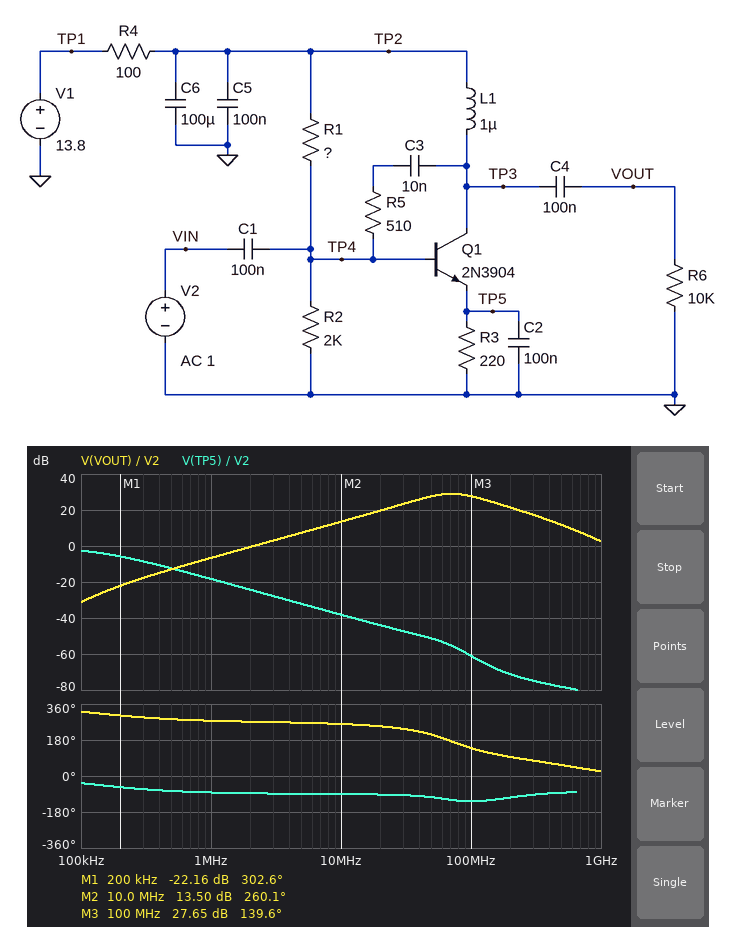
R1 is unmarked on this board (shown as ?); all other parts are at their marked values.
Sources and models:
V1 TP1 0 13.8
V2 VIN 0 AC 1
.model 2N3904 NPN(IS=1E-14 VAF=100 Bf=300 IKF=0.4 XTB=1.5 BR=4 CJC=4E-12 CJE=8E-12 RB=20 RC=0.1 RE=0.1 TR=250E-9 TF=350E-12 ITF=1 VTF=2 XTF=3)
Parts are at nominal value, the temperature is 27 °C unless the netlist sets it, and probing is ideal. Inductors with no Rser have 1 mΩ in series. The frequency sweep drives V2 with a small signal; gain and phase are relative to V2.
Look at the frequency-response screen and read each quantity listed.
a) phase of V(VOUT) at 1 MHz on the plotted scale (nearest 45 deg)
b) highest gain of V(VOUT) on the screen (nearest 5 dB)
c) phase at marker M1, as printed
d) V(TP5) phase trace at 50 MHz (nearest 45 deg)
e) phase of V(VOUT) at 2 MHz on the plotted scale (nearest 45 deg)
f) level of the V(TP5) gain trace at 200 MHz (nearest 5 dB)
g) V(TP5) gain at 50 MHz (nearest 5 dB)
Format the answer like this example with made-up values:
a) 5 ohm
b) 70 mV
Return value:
a) 270 deg
b) 30 dB
c) 302.6 deg
d) -90 deg
e) 270 deg
f) -70 dB
g) -50 dB
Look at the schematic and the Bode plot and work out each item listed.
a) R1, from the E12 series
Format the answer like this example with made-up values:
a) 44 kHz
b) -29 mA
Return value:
a) 22 kΩ
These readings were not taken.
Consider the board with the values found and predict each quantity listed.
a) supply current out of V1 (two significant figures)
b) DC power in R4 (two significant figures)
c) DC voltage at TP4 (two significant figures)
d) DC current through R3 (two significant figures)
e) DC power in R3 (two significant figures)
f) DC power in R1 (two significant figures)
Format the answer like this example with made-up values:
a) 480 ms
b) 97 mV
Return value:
a) 2.6 mA
b) 670 µW
c) 1.1 V
d) 2.0 mA
e) 910 µW
f) 7.0 mW
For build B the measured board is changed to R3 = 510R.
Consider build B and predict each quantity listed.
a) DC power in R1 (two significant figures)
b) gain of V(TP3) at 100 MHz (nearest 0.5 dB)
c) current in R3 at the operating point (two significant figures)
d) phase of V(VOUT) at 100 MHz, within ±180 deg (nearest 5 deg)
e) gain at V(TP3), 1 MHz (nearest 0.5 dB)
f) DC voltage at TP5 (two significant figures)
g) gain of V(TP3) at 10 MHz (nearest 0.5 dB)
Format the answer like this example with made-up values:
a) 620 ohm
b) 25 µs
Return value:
a) 7.1 mW
b) 23.0 dB
c) 940 µA
d) 160 deg
e) -13.5 dB
f) 480 mV
g) 6.5 dB
